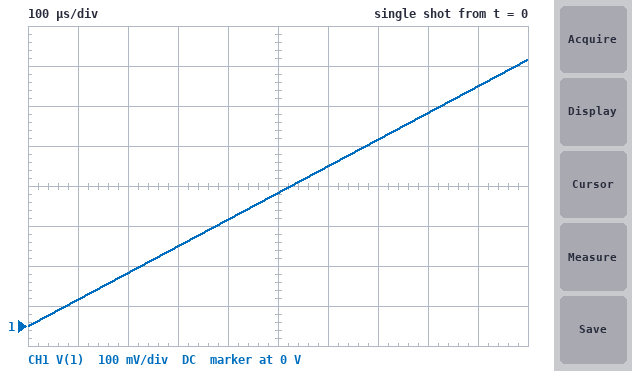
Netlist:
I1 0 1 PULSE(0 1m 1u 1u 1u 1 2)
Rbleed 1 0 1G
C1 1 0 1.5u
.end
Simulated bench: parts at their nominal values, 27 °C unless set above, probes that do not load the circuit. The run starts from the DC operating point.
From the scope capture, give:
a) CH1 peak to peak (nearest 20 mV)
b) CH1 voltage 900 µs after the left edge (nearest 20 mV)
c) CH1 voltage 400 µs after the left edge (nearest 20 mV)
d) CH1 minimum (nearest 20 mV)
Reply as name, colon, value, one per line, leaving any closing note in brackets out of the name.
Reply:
CH1 peak to peak: 660 mV
CH1 voltage 900 µs after the left edge: 600 mV
CH1 voltage 400 µs after the left edge: 260 mV
CH1 minimum: 0 V
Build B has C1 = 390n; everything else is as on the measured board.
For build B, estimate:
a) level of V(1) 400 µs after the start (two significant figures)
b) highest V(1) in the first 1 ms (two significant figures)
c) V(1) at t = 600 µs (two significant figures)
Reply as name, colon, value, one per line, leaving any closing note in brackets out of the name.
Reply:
level of V(1) 400 µs after the start: 1.0 V
highest V(1) in the first 1 ms: 2.6 V
V(1) at t = 600 µs: 1.5 V
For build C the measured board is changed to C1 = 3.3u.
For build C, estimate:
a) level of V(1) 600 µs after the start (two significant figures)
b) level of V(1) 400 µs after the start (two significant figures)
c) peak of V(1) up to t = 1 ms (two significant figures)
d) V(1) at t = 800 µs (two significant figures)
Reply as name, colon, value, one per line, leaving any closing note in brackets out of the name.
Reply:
level of V(1) 600 µs after the start: 180 mV
level of V(1) 400 µs after the start: 120 mV
peak of V(1) up to t = 1 ms: 300 mV
V(1) at t = 800 µs: 240 mV
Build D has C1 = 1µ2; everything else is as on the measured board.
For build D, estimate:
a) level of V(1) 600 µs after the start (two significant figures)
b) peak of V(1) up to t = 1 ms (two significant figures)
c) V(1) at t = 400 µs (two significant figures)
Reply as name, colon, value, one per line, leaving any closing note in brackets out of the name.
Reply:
level of V(1) 600 µs after the start: 500 mV
peak of V(1) up to t = 1 ms: 830 mV
V(1) at t = 400 µs: 330 mV
